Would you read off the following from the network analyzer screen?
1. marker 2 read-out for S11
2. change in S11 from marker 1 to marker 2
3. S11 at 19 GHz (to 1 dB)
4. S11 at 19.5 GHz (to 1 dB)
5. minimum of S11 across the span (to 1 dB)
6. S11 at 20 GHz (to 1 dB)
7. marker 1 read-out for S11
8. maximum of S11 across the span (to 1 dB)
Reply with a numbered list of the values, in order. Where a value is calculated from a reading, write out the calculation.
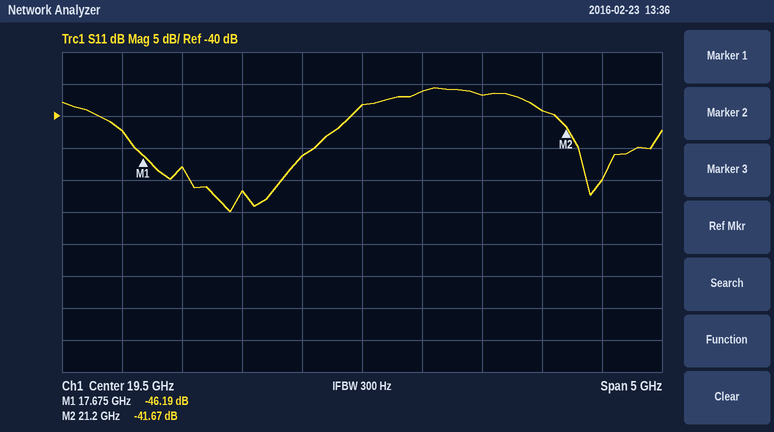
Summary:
1. -41.67 dB
2. -41.67 − (-46.19) = 4.52 dB
3. -46 dB
4. -38 dB
5. -55 dB
6. -36 dB
7. -46.19 dB
8. -36 dB
